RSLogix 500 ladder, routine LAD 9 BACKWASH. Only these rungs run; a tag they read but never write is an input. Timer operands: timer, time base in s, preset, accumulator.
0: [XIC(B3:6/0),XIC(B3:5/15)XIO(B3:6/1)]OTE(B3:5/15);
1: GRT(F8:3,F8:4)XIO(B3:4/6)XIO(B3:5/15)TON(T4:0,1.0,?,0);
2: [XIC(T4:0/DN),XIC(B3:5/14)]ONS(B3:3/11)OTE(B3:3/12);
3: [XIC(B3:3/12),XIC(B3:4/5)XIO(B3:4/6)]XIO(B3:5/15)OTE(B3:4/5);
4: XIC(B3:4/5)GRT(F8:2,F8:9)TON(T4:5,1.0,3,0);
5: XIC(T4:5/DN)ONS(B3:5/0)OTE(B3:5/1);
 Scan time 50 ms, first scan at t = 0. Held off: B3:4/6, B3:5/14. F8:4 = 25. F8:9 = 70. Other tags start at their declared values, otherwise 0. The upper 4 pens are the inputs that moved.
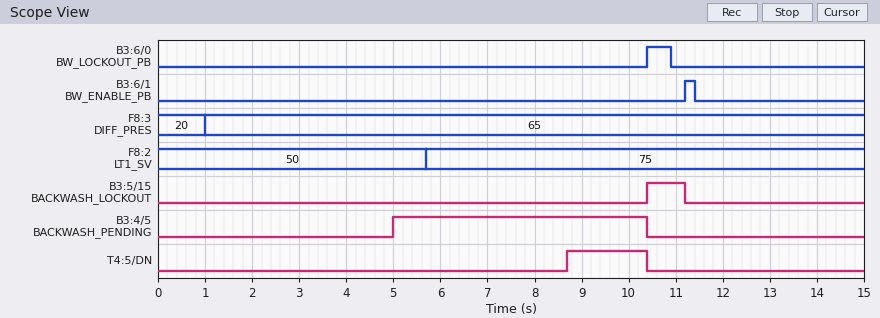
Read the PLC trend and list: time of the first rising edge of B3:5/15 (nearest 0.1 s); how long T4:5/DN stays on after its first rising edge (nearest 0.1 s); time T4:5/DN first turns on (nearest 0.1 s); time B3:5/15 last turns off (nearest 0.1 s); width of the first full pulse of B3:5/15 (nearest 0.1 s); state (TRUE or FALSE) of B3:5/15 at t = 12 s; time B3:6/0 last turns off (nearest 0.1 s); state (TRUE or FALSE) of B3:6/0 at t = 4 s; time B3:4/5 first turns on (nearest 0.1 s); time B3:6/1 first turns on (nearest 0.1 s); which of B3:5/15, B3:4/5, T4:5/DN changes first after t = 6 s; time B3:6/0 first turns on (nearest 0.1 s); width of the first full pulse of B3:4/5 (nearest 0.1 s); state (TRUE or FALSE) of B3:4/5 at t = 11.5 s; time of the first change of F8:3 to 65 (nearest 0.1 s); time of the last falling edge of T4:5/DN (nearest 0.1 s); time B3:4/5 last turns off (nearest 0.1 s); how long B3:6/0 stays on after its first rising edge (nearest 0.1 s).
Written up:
10.4 s
1.7 s
8.7 s
11.2 s
0.8 s
FALSE
10.9 s
FALSE
5.0 s
11.2 s
T4:5/DN
10.4 s
5.4 s
FALSE
1.0 s
10.4 s
10.4 s
0.5 s
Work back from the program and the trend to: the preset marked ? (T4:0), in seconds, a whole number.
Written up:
4 s
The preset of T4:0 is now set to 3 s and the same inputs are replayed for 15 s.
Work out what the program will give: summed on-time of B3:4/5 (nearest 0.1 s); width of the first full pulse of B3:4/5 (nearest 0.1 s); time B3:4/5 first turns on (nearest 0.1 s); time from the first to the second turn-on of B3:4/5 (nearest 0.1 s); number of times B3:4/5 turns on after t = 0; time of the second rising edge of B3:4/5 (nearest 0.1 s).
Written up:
7.2 s
6.4 s
4.0 s
10.2 s
2
14.2 s
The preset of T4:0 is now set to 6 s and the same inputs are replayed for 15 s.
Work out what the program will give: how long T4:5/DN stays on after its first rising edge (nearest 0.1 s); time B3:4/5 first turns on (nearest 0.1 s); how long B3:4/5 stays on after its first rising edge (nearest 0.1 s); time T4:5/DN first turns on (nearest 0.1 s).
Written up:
0.4 s
7.0 s
3.4 s
10.0 s
